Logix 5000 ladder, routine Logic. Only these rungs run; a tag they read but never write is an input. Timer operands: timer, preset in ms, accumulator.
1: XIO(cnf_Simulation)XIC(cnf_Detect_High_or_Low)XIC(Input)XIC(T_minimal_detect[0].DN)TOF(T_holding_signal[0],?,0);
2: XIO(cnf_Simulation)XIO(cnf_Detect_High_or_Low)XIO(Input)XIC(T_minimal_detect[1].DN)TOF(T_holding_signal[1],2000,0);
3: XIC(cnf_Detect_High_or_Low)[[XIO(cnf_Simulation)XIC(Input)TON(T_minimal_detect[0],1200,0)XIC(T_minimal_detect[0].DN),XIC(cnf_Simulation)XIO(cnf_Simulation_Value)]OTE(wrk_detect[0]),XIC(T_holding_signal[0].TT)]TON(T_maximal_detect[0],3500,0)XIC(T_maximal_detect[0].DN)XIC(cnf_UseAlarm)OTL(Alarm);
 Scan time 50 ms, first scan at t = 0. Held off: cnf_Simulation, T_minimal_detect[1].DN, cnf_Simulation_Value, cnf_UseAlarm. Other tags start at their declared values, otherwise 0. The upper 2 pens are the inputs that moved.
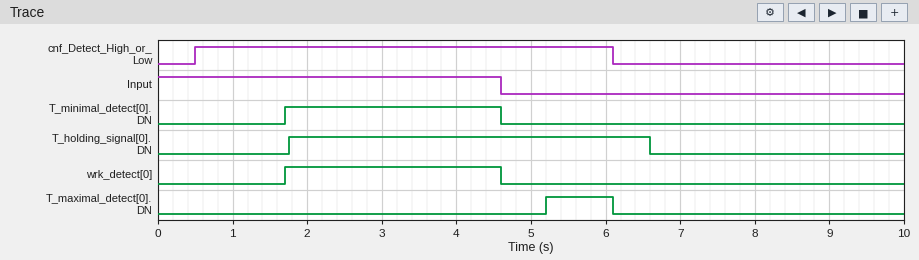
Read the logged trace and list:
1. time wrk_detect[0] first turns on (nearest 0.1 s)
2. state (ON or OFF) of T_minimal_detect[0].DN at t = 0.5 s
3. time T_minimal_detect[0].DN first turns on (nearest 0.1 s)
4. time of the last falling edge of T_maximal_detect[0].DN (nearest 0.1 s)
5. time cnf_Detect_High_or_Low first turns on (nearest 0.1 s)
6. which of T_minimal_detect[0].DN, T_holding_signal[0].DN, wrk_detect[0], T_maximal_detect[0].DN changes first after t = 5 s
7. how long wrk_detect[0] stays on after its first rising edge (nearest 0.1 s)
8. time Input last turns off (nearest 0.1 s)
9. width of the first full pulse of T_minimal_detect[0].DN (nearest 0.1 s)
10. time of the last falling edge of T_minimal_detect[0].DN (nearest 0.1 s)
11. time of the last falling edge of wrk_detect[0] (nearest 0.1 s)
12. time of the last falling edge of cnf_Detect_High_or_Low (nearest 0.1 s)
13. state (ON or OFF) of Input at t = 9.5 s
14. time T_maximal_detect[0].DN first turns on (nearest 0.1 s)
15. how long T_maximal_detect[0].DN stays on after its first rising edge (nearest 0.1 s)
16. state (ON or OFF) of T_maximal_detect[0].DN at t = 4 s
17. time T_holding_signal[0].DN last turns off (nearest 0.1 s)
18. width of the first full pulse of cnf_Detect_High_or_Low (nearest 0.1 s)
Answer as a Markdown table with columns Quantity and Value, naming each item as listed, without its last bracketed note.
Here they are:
| Quantity | Value |
|---|---|
| time wrk_detect[0] first turns on | 1.7 s |
| state (ON or OFF) of T_minimal_detect[0].DN at t = 0.5 s | OFF |
| time T_minimal_detect[0].DN first turns on | 1.7 s |
| time of the last falling edge of T_maximal_detect[0].DN | 6.1 s |
| time cnf_Detect_High_or_Low first turns on | 0.5 s |
| which of T_minimal_detect[0].DN, T_holding_signal[0].DN, wrk_detect[0], T_maximal_detect[0].DN changes first after t = 5 s | T_maximal_detect[0].DN |
| how long wrk_detect[0] stays on after its first rising edge | 2.9 s |
| time Input last turns off | 4.6 s |
| width of the first full pulse of T_minimal_detect[0].DN | 2.9 s |
| time of the last falling edge of T_minimal_detect[0].DN | 4.6 s |
| time of the last falling edge of wrk_detect[0] | 4.6 s |
| time of the last falling edge of cnf_Detect_High_or_Low | 6.1 s |
| state (ON or OFF) of Input at t = 9.5 s | OFF |
| time T_maximal_detect[0].DN first turns on | 5.2 s |
| how long T_maximal_detect[0].DN stays on after its first rising edge | 0.9 s |
| state (ON or OFF) of T_maximal_detect[0].DN at t = 4 s | OFF |
| time T_holding_signal[0].DN last turns off | 6.6 s |
| width of the first full pulse of cnf_Detect_High_or_Low | 5.6 s |
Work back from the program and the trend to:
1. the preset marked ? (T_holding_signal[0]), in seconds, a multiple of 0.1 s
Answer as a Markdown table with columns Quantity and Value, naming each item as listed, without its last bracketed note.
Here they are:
| Quantity | Value |
|---|---|
| the preset marked ? (T_holding_signal[0]), in seconds, a multiple of 0.1 s | 2.0 s |
